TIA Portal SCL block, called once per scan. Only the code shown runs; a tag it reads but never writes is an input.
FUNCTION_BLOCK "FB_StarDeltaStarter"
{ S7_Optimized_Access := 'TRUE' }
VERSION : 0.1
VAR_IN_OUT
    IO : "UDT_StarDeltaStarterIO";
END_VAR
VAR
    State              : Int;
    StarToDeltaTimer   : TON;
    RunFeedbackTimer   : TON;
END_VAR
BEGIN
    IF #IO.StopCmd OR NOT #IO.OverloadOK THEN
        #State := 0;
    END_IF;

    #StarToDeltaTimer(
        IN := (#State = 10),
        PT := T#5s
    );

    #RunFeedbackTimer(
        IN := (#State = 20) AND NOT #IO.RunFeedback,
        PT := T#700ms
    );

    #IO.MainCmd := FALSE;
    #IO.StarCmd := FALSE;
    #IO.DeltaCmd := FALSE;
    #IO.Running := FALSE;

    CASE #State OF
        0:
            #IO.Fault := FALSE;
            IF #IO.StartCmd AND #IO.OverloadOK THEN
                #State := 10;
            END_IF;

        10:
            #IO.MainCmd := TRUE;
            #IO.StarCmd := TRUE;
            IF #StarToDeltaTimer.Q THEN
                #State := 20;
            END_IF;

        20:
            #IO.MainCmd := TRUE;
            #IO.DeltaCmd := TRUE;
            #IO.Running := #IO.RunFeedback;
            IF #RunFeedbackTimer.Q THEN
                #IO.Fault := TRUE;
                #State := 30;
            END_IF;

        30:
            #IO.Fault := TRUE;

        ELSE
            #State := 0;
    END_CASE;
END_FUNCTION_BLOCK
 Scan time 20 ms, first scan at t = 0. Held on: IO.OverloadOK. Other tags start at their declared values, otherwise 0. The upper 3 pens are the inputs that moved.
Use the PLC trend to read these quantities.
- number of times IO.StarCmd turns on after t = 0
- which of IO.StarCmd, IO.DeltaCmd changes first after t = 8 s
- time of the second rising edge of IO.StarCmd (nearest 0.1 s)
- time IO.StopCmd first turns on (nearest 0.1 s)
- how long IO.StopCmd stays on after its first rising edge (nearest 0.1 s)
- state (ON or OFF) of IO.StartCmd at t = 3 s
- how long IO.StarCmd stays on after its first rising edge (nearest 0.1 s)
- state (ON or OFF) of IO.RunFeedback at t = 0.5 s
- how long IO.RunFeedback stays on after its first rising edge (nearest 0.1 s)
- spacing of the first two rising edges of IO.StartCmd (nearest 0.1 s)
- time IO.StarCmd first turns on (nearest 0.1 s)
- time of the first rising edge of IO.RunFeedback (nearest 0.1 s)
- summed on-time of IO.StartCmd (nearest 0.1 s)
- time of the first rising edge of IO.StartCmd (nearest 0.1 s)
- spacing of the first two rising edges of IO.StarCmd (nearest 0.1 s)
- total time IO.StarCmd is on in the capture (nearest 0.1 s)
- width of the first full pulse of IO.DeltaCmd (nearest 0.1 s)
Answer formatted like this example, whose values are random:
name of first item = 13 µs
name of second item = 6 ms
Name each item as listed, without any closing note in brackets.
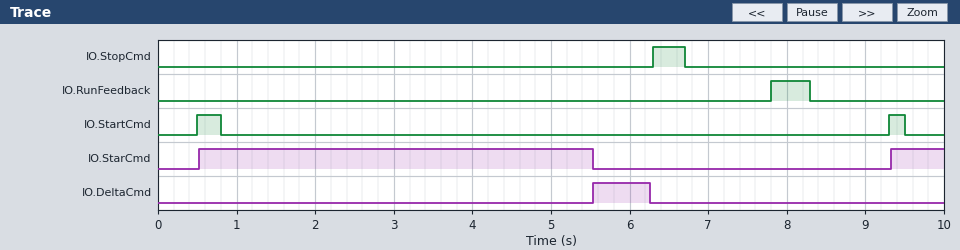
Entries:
number of times IO.StarCmd turns on after t = 0 = 2
which of IO.StarCmd, IO.DeltaCmd changes first after t = 8 s = IO.StarCmd
time of the second rising edge of IO.StarCmd = 9.3 s
time IO.StopCmd first turns on = 6.3 s
how long IO.StopCmd stays on after its first rising edge = 0.4 s
state (ON or OFF) of IO.StartCmd at t = 3 s = OFF
how long IO.StarCmd stays on after its first rising edge = 5.0 s
state (ON or OFF) of IO.RunFeedback at t = 0.5 s = OFF
how long IO.RunFeedback stays on after its first rising edge = 0.5 s
spacing of the first two rising edges of IO.StartCmd = 8.8 s
time IO.StarCmd first turns on = 0.5 s
time of the first rising edge of IO.RunFeedback = 7.8 s
summed on-time of IO.StartCmd = 0.5 s
time of the first rising edge of IO.StartCmd = 0.5 s
spacing of the first two rising edges of IO.StarCmd = 8.8 s
total time IO.StarCmd is on in the capture = 5.7 s
width of the first full pulse of IO.DeltaCmd = 0.7 s
